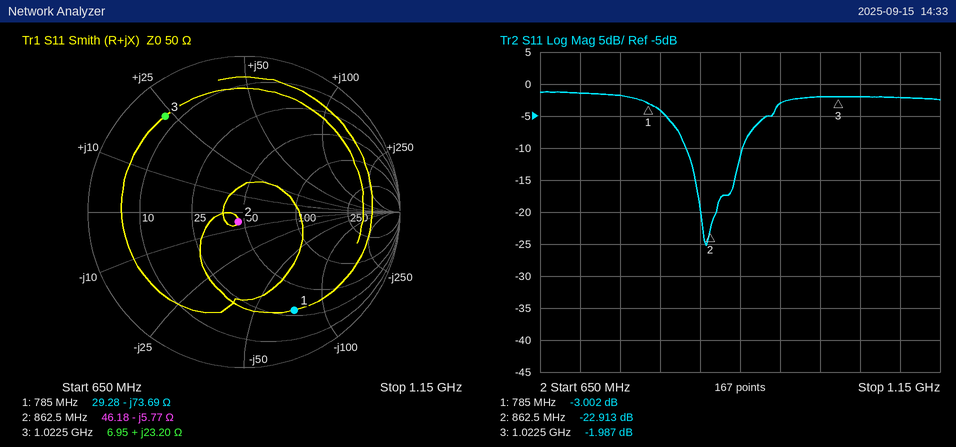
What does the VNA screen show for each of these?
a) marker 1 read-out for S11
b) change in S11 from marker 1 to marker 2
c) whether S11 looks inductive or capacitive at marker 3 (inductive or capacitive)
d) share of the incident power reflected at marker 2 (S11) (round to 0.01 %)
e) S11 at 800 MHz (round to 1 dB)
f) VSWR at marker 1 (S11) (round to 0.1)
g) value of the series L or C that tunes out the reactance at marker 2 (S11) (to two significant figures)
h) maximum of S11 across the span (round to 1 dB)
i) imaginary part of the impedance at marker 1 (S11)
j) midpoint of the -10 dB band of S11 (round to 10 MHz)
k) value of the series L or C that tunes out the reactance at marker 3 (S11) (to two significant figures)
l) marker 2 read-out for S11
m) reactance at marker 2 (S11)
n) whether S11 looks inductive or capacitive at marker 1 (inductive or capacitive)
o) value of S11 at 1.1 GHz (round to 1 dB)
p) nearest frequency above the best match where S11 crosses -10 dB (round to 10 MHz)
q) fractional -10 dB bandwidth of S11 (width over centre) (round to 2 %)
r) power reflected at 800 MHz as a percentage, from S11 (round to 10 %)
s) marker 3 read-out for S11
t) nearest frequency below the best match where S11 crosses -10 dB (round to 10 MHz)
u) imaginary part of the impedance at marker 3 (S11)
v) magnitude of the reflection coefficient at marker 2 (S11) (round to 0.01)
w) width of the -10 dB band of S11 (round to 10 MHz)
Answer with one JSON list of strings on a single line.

["-3.002 dB", "-19.911 dB", "inductive", "0.51 %", "-4 dB", "5.8", "1.1 nH", "-1 dB", "-73.69 Ω", "870 MHz", "6.7 pF", "-22.913 dB", "-5.77 Ω", "capacitive", "-2 dB", "900 MHz", "8 %", "40 %", "-1.987 dB", "830 MHz", "+23.20 Ω", "0.07", "70 MHz"]
